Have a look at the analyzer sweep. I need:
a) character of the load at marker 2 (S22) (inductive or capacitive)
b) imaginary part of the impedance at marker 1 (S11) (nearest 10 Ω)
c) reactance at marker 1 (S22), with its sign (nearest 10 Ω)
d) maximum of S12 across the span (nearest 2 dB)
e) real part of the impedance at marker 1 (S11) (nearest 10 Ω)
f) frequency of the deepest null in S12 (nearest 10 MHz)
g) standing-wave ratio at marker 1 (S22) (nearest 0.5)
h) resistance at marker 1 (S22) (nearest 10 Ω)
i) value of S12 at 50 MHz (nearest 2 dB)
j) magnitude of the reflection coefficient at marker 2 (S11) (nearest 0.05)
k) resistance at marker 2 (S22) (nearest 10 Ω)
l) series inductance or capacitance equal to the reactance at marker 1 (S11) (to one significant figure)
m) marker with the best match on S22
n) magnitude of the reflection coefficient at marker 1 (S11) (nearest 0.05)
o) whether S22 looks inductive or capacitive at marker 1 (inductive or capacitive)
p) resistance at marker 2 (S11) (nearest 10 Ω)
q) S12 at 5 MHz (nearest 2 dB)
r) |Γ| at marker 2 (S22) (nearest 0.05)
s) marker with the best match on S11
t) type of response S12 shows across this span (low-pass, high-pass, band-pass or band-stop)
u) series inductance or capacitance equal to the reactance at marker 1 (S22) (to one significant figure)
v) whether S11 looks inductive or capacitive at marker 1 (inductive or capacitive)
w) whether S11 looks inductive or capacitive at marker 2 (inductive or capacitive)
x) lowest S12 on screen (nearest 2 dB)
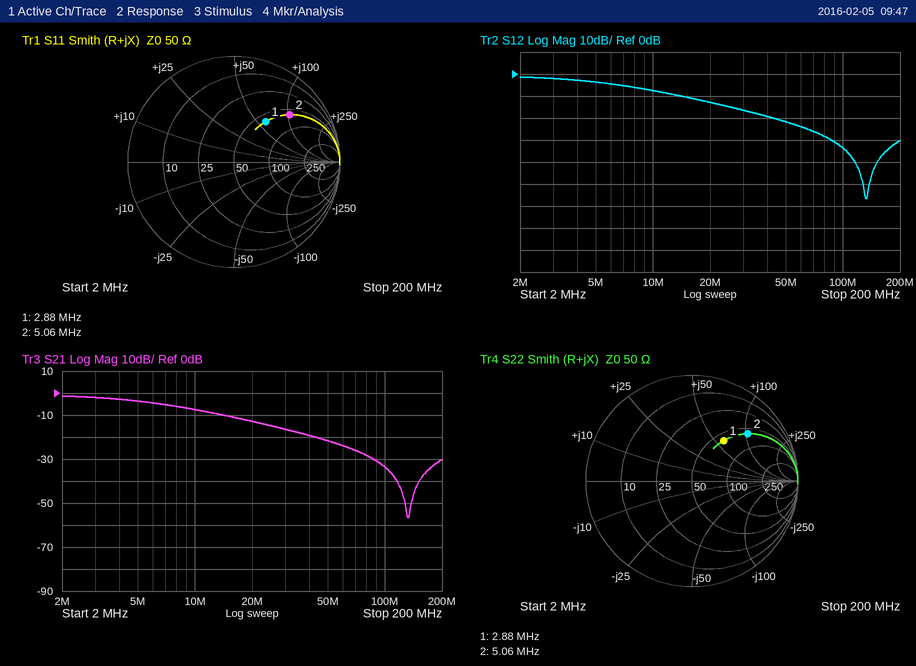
inductive
+60 Ω
+60 Ω
-2 dB
60 Ω
130 MHz
3.0
60 Ω
-22 dB
0.70
60 Ω
3 µH
marker 1
0.50
inductive
60 Ω
-4 dB
0.70
marker 1
low-pass
3 µH
inductive
inductive
-56 dB
